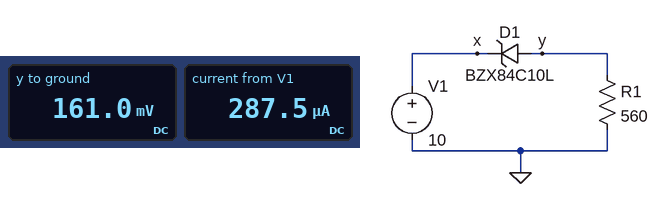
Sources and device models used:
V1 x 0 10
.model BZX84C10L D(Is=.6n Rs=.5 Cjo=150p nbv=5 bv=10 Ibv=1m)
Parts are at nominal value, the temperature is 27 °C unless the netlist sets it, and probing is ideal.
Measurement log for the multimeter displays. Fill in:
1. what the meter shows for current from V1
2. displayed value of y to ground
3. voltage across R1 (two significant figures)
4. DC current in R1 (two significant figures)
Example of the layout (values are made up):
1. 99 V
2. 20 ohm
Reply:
1. 287.5 µA
2. 161.0 mV
3. 160 mV
4. 290 µA
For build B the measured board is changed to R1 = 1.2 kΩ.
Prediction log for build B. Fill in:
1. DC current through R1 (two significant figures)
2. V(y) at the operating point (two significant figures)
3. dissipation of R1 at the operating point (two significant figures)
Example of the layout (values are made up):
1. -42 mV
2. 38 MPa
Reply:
1. 180 µA
2. 220 mV
3. 40 µW
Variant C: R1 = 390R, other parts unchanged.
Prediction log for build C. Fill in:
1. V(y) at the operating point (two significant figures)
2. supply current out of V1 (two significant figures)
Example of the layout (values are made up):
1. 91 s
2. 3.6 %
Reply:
1. 140 mV
2. 350 µA
